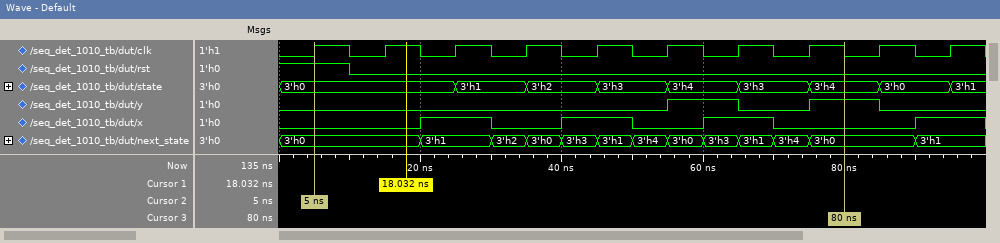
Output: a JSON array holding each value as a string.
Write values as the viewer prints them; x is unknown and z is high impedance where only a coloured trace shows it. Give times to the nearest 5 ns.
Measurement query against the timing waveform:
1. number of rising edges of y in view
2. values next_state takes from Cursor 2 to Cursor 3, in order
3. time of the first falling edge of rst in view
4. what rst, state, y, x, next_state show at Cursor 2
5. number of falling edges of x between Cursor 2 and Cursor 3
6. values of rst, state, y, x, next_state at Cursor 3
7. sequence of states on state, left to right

["2", "3'h0, 3'h1, 3'h2, 3'h0, 3'h3, 3'h1, 3'h4, 3'h0, 3'h3, 3'h1, 3'h4, 3'h0", "10 ns", "rst=1, state=3'h0, y=0, x=0, next_state=3'h0", "3", "rst=0, state=3'h4, y=1, x=0, next_state=3'h0", "3'h0, 3'h1, 3'h2, 3'h3, 3'h4, 3'h3, 3'h4, 3'h0, 3'h1"]
